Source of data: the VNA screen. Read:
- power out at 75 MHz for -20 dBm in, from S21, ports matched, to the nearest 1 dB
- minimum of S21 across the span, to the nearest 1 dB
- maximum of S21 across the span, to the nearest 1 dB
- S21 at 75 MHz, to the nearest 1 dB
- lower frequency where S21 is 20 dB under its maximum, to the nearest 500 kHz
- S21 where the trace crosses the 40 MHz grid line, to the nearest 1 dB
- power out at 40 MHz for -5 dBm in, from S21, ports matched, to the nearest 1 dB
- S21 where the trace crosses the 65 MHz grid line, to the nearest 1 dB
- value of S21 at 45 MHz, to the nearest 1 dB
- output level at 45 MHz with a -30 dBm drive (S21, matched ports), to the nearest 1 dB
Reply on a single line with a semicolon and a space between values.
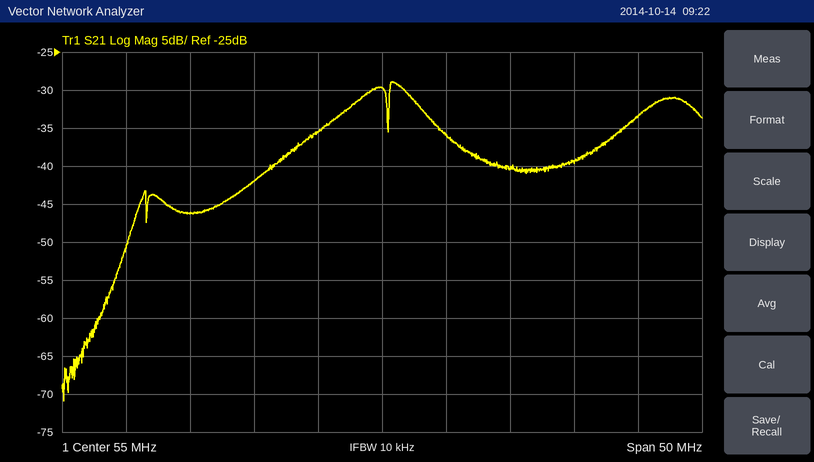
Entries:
-53 dBm; -71 dB; -29 dB; -33 dB; 35.5 MHz; -46 dB; -51 dBm; -40 dB; -42 dB; -72 dBm
